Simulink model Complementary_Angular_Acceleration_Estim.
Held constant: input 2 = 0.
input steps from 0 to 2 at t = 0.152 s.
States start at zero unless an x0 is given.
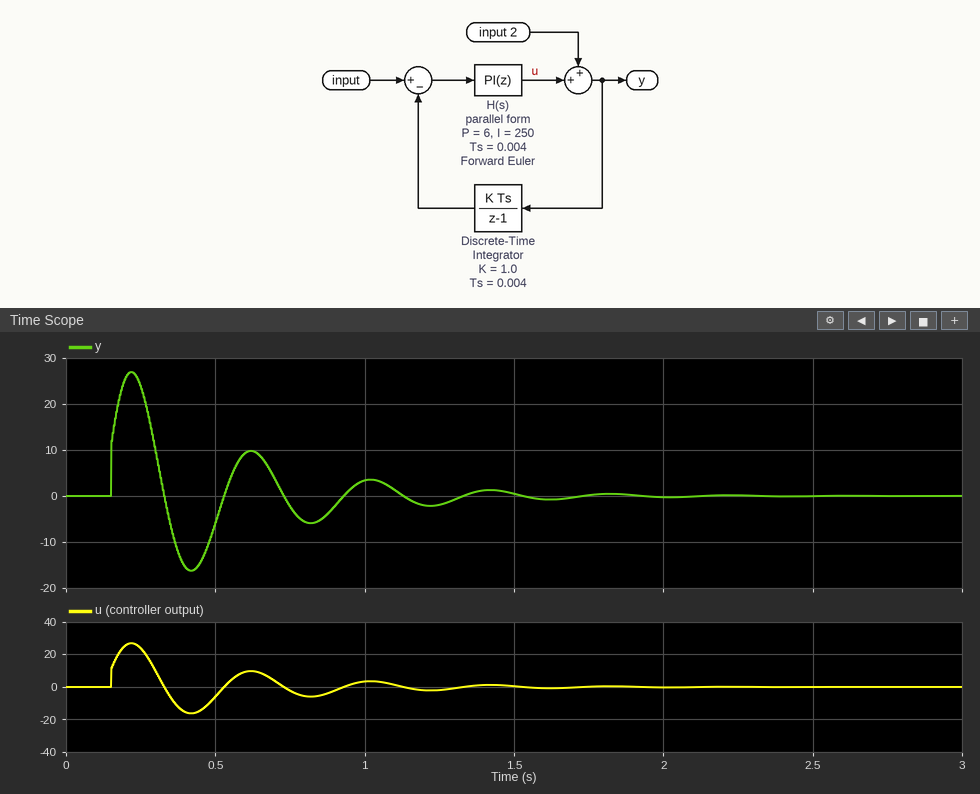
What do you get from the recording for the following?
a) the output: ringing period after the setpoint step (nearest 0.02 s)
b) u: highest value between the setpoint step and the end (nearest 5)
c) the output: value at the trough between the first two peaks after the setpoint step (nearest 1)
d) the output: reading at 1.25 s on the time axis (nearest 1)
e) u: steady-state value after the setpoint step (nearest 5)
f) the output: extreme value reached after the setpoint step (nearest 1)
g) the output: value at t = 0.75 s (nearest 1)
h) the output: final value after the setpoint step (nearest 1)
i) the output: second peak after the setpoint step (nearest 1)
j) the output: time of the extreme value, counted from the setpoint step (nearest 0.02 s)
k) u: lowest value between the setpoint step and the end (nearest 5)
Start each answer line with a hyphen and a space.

- 0.40 s
- 25
- -16
- -2
- 0
- 27
- -2
- 0
- 10
- 0.06 s
- -15
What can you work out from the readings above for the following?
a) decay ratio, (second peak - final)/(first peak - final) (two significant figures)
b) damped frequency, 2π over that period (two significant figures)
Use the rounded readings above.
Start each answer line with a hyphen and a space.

- 0.37
- 16 rad/s
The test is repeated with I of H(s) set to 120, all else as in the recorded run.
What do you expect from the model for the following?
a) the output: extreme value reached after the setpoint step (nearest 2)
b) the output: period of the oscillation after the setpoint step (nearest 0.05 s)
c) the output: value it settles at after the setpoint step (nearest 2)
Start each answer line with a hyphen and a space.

- 18
- 0.60 s
- 0
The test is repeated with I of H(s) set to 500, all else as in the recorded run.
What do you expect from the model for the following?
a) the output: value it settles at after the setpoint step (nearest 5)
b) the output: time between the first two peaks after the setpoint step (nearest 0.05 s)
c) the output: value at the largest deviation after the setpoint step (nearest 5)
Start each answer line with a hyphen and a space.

- 0
- 0.30 s
- 40
